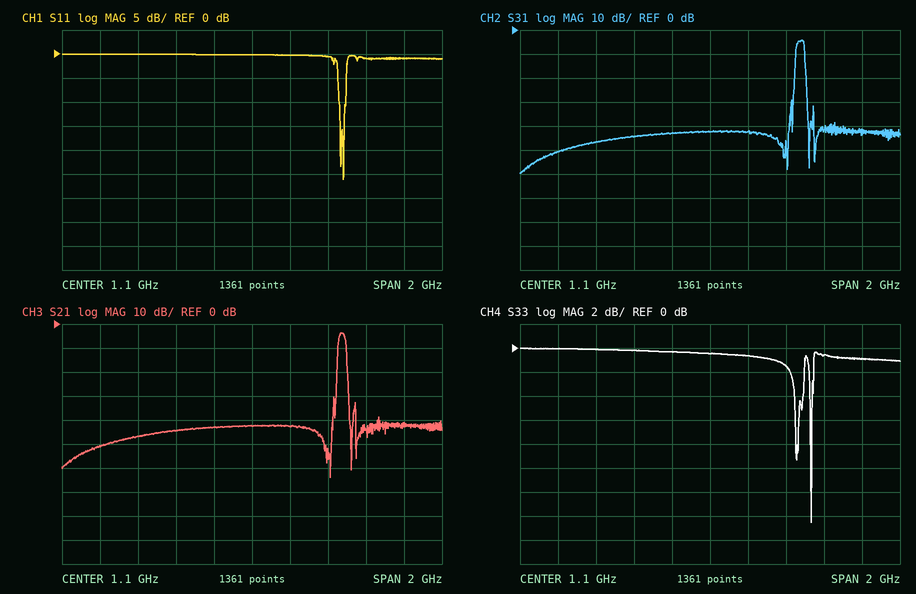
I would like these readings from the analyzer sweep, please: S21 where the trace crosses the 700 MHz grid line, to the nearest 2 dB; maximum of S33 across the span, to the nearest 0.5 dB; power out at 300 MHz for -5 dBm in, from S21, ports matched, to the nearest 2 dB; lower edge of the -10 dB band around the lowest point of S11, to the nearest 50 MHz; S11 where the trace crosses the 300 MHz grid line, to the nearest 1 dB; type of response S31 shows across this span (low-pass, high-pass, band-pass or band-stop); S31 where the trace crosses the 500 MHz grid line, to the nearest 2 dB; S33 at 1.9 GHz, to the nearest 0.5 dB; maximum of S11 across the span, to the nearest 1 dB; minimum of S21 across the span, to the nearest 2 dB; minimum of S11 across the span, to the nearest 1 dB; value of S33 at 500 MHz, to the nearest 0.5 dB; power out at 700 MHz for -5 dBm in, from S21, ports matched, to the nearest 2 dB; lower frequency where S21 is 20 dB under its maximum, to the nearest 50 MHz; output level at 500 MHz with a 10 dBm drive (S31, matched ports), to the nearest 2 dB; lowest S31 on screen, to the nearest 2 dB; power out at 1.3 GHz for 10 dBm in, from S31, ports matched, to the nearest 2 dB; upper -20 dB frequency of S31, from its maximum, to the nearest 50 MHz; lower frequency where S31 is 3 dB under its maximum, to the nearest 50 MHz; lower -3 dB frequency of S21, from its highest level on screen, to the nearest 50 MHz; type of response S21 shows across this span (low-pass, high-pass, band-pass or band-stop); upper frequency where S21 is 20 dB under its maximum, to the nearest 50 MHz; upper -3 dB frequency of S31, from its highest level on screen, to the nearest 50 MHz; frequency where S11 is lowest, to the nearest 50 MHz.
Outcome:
-44 dB
0.0 dB
-56 dBm
1.55 GHz
0 dB
band-pass
-46 dB
-1.0 dB
0 dB
-64 dB
-26 dB
0.0 dB
-50 dBm
1.55 GHz
-36 dBm
-60 dB
-32 dBm
1.60 GHz
1.55 GHz
1.55 GHz
band-pass
1.60 GHz
1.60 GHz
1.60 GHz
